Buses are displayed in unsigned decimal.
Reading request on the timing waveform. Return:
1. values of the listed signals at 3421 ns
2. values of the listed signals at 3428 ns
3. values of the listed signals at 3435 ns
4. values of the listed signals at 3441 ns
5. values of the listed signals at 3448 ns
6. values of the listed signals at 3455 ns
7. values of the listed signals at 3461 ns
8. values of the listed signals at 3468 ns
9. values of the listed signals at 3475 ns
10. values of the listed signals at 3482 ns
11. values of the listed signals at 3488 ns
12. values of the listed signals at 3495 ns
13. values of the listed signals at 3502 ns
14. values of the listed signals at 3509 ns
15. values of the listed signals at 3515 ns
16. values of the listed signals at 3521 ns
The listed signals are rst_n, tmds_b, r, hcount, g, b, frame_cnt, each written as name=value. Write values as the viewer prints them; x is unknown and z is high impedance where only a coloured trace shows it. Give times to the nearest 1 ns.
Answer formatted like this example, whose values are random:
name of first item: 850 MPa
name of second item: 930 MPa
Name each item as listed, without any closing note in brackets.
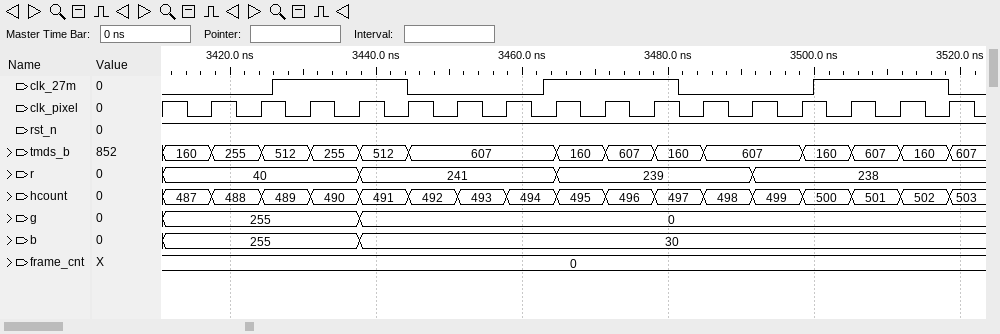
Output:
values of the listed signals at 3421 ns: rst_n=1, tmds_b=255, r=40, hcount=488, g=255, b=255, frame_cnt=0
values of the listed signals at 3428 ns: rst_n=1, tmds_b=512, r=40, hcount=489, g=255, b=255, frame_cnt=0
values of the listed signals at 3435 ns: rst_n=1, tmds_b=255, r=40, hcount=490, g=255, b=255, frame_cnt=0
values of the listed signals at 3441 ns: rst_n=1, tmds_b=512, r=241, hcount=491, g=0, b=30, frame_cnt=0
values of the listed signals at 3448 ns: rst_n=1, tmds_b=607, r=241, hcount=492, g=0, b=30, frame_cnt=0
values of the listed signals at 3455 ns: rst_n=1, tmds_b=607, r=241, hcount=493, g=0, b=30, frame_cnt=0
values of the listed signals at 3461 ns: rst_n=1, tmds_b=607, r=241, hcount=494, g=0, b=30, frame_cnt=0
values of the listed signals at 3468 ns: rst_n=1, tmds_b=160, r=239, hcount=495, g=0, b=30, frame_cnt=0
values of the listed signals at 3475 ns: rst_n=1, tmds_b=607, r=239, hcount=496, g=0, b=30, frame_cnt=0
values of the listed signals at 3482 ns: rst_n=1, tmds_b=160, r=239, hcount=497, g=0, b=30, frame_cnt=0
values of the listed signals at 3488 ns: rst_n=1, tmds_b=607, r=239, hcount=498, g=0, b=30, frame_cnt=0
values of the listed signals at 3495 ns: rst_n=1, tmds_b=607, r=238, hcount=499, g=0, b=30, frame_cnt=0
values of the listed signals at 3502 ns: rst_n=1, tmds_b=160, r=238, hcount=500, g=0, b=30, frame_cnt=0
values of the listed signals at 3509 ns: rst_n=1, tmds_b=607, r=238, hcount=501, g=0, b=30, frame_cnt=0
values of the listed signals at 3515 ns: rst_n=1, tmds_b=160, r=238, hcount=502, g=0, b=30, frame_cnt=0
values of the listed signals at 3521 ns: rst_n=1, tmds_b=607, r=238, hcount=503, g=0, b=30, frame_cnt=0
